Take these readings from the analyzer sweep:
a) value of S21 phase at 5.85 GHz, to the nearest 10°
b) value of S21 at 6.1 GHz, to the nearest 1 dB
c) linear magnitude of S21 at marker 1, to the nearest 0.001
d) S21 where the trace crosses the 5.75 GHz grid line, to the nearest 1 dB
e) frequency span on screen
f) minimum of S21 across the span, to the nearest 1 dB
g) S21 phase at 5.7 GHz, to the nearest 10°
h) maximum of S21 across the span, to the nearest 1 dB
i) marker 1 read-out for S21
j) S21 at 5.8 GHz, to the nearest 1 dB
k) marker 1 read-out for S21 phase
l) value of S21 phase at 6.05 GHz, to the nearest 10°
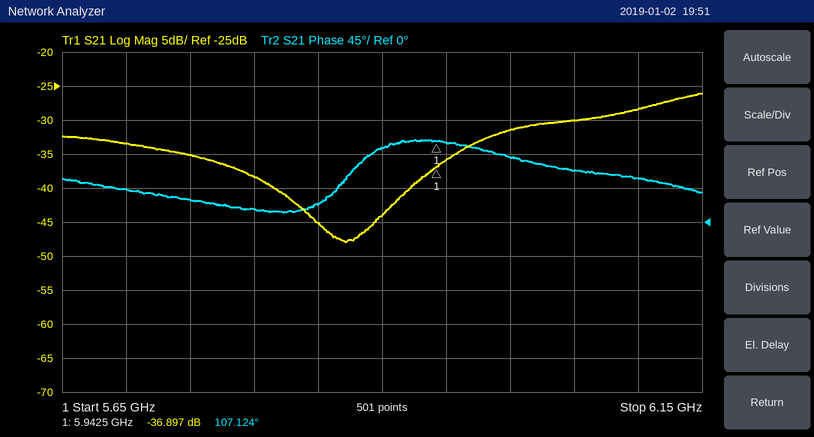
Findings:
20°
-28 dB
0.014
-35 dB
500 MHz
-48 dB
40°
-26 dB
-36.897 dB
-38 dB
107.124°
70°
